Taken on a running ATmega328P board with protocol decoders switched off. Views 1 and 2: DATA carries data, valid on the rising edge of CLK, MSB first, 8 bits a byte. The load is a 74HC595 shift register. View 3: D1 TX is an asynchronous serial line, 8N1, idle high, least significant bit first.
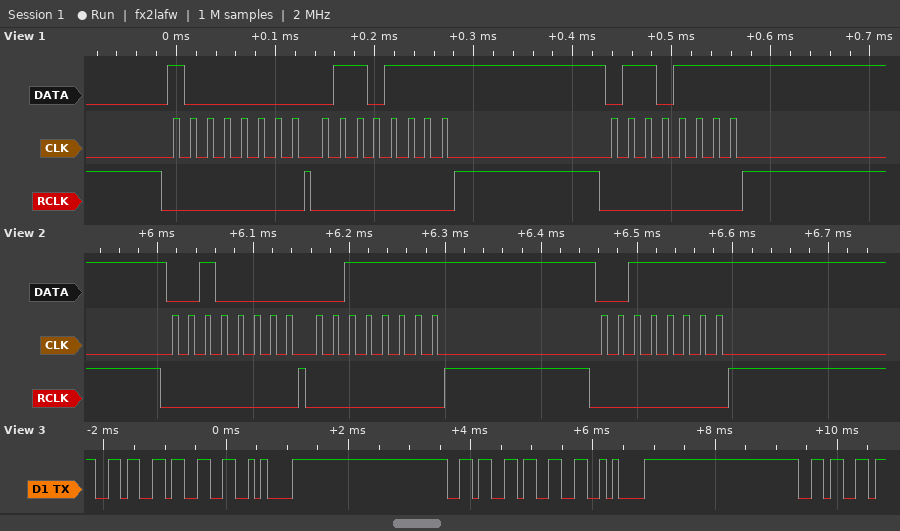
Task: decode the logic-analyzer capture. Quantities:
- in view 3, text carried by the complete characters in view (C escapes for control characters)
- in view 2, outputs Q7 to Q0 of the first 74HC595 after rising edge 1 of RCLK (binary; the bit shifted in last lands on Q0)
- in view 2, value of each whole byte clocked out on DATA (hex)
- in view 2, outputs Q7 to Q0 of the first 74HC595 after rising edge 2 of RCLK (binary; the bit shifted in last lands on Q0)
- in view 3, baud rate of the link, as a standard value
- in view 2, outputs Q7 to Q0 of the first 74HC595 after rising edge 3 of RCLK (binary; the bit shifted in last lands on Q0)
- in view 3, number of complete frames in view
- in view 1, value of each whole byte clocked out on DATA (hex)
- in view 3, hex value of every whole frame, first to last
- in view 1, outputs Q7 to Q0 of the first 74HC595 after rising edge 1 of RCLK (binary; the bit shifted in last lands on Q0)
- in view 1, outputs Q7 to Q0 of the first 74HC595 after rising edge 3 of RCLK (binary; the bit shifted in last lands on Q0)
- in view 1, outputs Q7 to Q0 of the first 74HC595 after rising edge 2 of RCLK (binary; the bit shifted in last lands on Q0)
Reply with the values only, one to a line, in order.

"63\n63\n6"
00100000
20 3F 3F
00111111
9600 baud
00111111
7
80 6F 6F
0x36 0x33 0x0A 0x36 0x33 0x0A 0x36
10000000
01101111
01101111
